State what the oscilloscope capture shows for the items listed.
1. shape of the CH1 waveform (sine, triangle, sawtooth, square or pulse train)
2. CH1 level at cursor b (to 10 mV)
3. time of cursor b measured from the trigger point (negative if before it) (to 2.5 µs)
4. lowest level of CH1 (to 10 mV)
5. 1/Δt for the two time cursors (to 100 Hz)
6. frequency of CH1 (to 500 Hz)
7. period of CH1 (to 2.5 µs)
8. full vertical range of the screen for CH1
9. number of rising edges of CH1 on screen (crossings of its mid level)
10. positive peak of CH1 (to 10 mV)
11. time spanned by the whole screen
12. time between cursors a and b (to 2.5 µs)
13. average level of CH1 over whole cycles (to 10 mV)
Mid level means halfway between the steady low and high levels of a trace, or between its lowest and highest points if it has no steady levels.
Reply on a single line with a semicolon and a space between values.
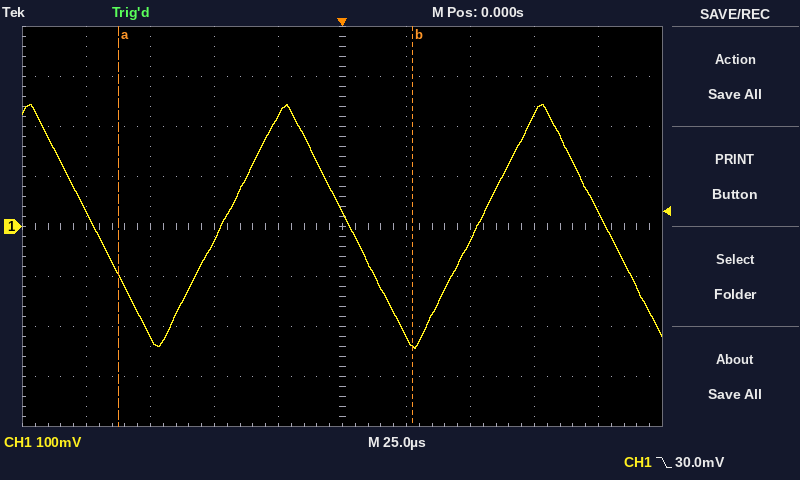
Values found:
triangle; -240 mV; +27.5 µs; -240 mV; 8.7 kHz; 10.0 kHz; 100.0 µs; 800 mV; 2; 240 mV; 250 µs; 115.0 µs; 0 mV
